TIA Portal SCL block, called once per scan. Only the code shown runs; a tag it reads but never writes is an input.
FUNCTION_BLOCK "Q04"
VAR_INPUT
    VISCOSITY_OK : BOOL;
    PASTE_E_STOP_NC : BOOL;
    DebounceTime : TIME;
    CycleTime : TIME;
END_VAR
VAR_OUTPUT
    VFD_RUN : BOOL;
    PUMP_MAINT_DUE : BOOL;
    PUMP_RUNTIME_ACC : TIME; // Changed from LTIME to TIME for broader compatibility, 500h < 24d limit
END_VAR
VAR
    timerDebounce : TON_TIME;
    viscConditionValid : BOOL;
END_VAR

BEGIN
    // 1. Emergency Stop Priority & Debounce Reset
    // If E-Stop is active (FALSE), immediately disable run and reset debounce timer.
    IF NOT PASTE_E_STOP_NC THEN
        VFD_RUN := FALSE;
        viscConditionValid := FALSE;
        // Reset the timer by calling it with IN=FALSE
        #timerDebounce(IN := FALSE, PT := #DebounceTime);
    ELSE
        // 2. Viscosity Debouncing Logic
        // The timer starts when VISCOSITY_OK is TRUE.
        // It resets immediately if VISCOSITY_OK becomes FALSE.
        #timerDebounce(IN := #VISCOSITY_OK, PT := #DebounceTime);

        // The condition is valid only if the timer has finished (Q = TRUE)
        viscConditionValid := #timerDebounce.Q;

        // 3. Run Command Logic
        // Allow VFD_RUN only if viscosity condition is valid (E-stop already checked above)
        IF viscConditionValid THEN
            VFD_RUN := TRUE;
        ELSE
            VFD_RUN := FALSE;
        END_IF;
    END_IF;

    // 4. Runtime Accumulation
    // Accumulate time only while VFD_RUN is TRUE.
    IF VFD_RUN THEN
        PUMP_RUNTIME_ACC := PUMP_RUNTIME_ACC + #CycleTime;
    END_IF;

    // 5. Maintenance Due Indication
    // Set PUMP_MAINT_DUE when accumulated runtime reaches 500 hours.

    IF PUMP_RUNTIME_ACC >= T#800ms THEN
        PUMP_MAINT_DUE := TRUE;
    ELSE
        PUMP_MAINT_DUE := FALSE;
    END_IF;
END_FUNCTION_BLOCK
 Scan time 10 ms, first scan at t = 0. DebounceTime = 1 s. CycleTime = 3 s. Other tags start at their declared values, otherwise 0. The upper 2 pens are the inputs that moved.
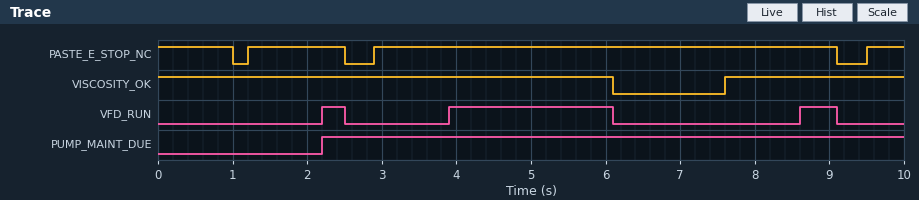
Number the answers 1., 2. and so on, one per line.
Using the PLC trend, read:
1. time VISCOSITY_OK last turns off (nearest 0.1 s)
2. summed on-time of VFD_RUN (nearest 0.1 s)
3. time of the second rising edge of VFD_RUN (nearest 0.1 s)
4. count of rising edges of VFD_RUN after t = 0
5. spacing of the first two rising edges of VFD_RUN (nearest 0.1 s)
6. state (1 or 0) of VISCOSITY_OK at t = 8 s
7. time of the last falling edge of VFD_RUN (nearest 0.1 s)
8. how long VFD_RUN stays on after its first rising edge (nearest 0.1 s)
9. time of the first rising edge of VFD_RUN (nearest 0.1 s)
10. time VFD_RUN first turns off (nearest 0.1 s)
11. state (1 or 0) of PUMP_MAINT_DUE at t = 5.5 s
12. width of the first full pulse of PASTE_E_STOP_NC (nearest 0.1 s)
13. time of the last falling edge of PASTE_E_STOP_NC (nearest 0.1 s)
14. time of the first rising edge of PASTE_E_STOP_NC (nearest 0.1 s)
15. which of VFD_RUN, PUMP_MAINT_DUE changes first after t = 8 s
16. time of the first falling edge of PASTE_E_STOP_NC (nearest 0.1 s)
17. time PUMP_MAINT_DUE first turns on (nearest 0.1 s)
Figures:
1. 6.1 s
2. 3.0 s
3. 3.9 s
4. 3
5. 1.7 s
6. 1
7. 9.1 s
8. 0.3 s
9. 2.2 s
10. 2.5 s
11. 1
12. 1.3 s
13. 9.1 s
14. 1.2 s
15. VFD_RUN
16. 1.0 s
17. 2.2 s
